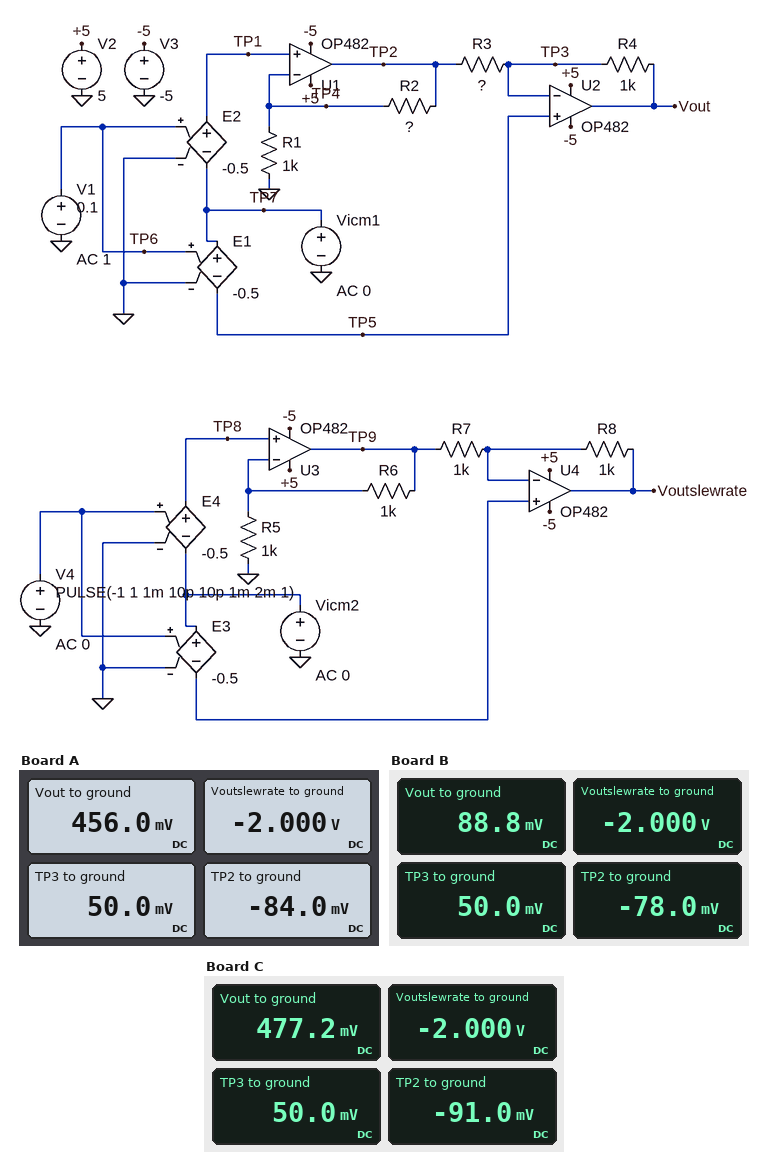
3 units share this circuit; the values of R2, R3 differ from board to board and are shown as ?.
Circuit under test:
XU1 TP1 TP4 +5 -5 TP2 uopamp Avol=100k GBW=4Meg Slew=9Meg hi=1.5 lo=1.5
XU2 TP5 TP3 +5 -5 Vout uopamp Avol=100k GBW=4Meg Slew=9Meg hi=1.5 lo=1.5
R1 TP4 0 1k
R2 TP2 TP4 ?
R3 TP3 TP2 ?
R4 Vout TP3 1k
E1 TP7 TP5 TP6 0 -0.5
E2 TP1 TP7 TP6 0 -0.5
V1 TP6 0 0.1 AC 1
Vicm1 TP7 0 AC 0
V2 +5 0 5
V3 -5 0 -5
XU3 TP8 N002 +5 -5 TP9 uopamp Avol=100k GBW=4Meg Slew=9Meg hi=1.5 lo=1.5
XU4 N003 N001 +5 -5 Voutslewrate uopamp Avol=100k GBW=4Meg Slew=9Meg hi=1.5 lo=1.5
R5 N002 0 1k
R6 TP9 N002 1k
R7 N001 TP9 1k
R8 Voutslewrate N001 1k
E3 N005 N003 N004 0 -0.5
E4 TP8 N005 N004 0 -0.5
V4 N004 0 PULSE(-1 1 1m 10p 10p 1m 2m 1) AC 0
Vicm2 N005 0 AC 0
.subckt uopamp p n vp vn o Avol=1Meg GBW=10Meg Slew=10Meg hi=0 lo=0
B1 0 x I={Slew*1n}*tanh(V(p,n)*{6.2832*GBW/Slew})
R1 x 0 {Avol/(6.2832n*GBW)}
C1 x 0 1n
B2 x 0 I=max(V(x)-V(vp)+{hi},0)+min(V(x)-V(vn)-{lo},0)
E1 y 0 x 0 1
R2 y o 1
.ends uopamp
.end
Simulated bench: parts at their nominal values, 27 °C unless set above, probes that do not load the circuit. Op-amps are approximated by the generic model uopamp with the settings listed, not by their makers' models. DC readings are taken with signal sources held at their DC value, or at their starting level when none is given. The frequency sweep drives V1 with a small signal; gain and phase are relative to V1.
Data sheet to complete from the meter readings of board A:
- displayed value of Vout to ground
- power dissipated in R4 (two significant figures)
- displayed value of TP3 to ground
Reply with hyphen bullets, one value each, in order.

- 456.0 mV
- 160 µW
- 50.0 mV
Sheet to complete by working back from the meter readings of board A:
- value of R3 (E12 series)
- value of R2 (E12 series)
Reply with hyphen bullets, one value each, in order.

- 330 Ω
- 680 Ω
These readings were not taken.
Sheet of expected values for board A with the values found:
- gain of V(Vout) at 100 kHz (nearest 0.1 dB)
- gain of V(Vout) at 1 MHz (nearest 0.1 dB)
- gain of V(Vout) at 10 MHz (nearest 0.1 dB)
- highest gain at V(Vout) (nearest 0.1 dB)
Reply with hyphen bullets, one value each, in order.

- 13.1 dB
- 9.6 dB
- -13.2 dB
- 13.2 dB
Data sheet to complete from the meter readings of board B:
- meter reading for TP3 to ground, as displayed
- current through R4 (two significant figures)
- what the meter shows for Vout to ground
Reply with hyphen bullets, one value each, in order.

- 50.0 mV
- 39 µA
- 88.8 mV
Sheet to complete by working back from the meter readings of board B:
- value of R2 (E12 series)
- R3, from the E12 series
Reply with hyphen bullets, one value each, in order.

- 560 Ω
- 3.3 kΩ
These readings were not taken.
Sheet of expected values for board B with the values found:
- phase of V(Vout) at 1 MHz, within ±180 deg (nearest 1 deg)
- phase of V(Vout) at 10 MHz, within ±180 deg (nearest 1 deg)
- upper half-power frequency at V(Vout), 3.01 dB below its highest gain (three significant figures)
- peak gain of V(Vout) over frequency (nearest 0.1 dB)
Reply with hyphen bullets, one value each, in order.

- -23 deg
- -78 deg
- 2.34 MHz
- -1.0 dB
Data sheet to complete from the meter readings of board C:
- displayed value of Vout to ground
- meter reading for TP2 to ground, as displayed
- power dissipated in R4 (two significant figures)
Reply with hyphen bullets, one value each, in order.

- 477.2 mV
- -91.0 mV
- 180 µW
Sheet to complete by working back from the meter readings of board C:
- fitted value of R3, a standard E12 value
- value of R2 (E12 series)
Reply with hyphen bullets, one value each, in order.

- 330 Ω
- 820 Ω
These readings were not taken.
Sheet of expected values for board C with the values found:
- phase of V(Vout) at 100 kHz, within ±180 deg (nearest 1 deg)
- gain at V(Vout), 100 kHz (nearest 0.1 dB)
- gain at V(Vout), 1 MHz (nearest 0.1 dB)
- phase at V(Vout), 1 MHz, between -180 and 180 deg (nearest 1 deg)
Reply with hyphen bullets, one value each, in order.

- -7 deg
- 13.5 dB
- 9.9 dB
- -59 deg
